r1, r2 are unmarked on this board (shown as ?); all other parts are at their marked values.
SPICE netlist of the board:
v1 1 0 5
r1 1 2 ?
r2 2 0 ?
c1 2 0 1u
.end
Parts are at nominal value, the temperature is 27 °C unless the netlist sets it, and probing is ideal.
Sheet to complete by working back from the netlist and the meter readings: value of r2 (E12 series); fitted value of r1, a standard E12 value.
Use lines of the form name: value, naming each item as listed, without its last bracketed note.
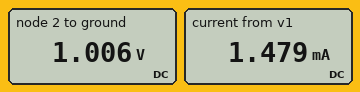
value of r2: 680 Ω
fitted value of r1, a standard E12 value: 2.7 kΩ
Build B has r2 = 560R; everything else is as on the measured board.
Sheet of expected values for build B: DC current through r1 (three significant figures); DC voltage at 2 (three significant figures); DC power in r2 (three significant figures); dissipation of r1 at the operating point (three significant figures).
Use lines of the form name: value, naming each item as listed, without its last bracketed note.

DC current through r1: 1.53 mA
DC voltage at 2: 859 mV
DC power in r2: 1.32 mW
dissipation of r1 at the operating point: 6.35 mW
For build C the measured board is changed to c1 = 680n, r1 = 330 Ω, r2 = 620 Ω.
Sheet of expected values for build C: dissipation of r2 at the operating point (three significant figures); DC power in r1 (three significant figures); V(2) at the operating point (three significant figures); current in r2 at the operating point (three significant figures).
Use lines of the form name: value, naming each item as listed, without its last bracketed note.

dissipation of r2 at the operating point: 17.2 mW
DC power in r1: 9.14 mW
V(2) at the operating point: 3.26 V
current in r2 at the operating point: 5.26 mA
